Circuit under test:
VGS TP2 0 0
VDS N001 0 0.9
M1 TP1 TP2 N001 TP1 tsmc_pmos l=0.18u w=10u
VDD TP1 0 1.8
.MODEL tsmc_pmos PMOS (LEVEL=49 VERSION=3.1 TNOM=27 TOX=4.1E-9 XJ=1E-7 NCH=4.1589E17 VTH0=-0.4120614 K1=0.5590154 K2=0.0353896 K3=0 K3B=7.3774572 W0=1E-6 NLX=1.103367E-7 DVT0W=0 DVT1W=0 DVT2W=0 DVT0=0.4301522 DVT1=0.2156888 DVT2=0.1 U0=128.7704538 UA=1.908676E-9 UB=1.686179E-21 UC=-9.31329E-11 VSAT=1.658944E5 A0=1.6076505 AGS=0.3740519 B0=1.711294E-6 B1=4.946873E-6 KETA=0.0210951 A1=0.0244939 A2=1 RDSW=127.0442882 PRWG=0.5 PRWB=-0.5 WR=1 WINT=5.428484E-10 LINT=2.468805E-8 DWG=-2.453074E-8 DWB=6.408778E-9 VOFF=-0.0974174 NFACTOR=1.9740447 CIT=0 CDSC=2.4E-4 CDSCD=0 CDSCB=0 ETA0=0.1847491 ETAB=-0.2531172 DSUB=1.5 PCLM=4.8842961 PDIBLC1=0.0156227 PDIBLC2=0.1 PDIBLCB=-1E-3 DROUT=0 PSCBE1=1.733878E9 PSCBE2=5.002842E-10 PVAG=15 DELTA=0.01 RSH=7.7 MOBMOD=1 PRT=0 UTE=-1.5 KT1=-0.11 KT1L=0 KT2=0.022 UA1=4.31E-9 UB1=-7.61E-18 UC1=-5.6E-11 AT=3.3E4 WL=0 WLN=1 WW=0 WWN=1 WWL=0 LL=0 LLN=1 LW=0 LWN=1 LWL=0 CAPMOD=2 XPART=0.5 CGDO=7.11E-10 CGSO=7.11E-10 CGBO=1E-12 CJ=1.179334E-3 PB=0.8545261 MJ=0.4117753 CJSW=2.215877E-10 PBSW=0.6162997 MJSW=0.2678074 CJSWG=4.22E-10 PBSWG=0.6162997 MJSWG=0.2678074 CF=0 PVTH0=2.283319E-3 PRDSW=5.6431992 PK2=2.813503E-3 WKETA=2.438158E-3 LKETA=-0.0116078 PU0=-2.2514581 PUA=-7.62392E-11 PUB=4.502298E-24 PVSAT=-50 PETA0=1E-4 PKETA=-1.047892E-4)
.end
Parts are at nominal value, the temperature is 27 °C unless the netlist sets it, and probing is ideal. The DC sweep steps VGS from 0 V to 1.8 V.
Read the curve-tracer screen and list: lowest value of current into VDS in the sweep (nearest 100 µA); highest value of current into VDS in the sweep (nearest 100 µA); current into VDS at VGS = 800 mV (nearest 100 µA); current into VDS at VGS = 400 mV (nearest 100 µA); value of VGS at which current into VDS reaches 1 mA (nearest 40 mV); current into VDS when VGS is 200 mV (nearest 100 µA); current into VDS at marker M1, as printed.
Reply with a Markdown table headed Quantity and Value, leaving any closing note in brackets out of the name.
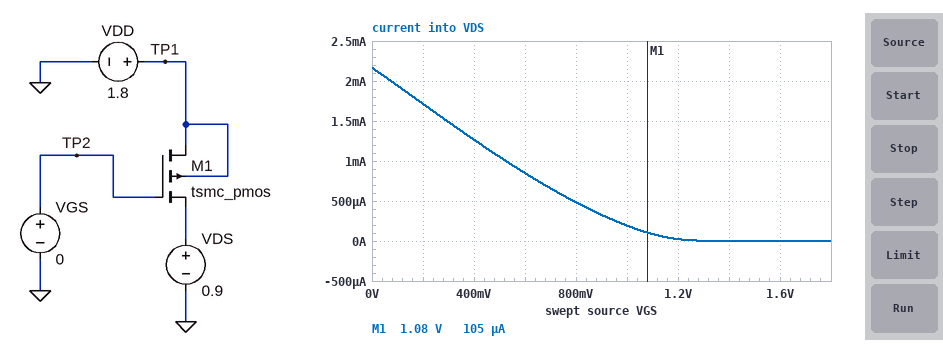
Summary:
| Quantity | Value |
|---|---|
| lowest value of current into VDS in the sweep | 0 A |
| highest value of current into VDS in the sweep | 2.2 mA |
| current into VDS at VGS = 800 mV | 500 µA |
| current into VDS at VGS = 400 mV | 1.3 mA |
| value of VGS at which current into VDS reaches 1 mA | 520 mV |
| current into VDS when VGS is 200 mV | 1.7 mA |
| current into VDS at marker M1, as printed | 105 µA |
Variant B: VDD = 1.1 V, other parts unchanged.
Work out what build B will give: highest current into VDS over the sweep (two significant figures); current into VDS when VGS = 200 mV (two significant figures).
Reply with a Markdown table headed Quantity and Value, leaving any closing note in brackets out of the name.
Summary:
| Quantity | Value |
|---|---|
| highest current into VDS over the sweep | 390 µA |
| current into VDS when VGS = 200 mV | 240 µA |
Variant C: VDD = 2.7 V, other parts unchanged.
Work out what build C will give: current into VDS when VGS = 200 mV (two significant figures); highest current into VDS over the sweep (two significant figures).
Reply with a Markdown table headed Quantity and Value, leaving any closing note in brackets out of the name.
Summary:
| Quantity | Value |
|---|---|
| current into VDS when VGS = 200 mV | 4.4 mA |
| highest current into VDS over the sweep | 5.0 mA |
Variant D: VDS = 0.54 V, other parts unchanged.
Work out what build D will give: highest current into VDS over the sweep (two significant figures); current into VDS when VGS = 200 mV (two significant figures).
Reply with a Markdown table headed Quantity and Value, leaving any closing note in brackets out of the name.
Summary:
| Quantity | Value |
|---|---|
| highest current into VDS over the sweep | 2.3 mA |
| current into VDS when VGS = 200 mV | 1.8 mA |
